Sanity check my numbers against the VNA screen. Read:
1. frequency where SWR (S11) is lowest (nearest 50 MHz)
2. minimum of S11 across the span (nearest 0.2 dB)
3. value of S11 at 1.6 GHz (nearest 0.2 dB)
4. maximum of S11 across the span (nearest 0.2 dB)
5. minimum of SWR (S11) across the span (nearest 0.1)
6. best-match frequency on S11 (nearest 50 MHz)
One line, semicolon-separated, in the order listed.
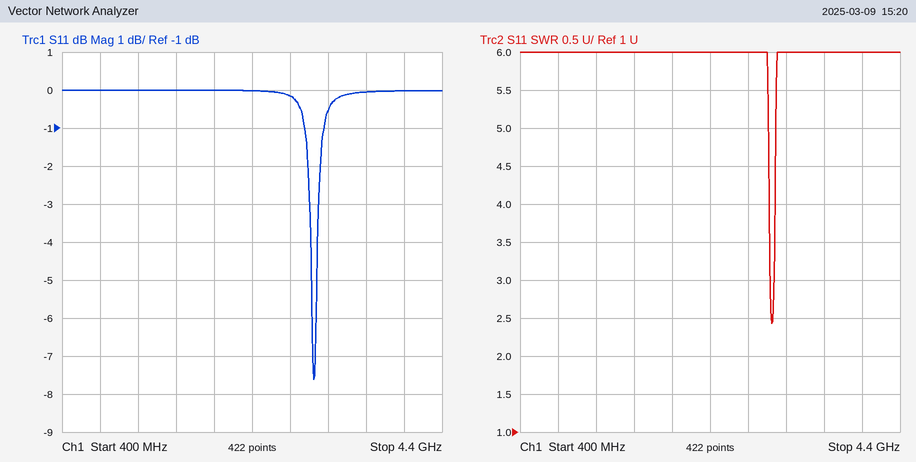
3.05 GHz; -7.6 dB; 0.0 dB; 0.0 dB; 2.4; 3.05 GHz
